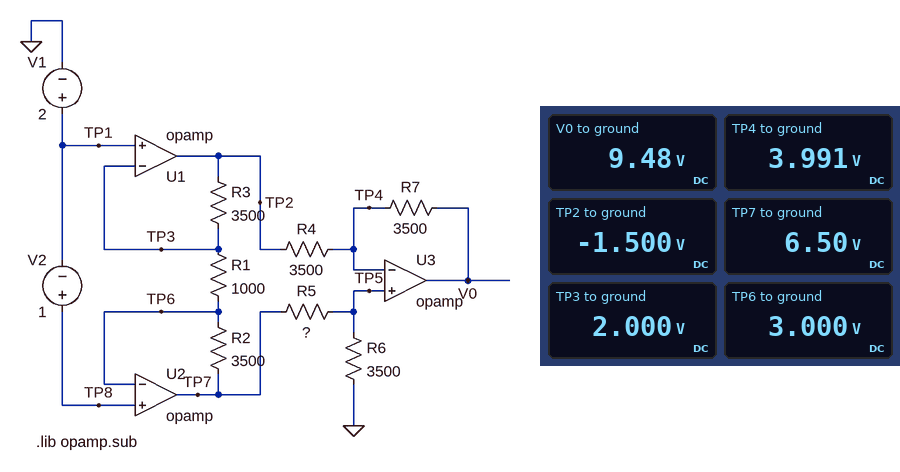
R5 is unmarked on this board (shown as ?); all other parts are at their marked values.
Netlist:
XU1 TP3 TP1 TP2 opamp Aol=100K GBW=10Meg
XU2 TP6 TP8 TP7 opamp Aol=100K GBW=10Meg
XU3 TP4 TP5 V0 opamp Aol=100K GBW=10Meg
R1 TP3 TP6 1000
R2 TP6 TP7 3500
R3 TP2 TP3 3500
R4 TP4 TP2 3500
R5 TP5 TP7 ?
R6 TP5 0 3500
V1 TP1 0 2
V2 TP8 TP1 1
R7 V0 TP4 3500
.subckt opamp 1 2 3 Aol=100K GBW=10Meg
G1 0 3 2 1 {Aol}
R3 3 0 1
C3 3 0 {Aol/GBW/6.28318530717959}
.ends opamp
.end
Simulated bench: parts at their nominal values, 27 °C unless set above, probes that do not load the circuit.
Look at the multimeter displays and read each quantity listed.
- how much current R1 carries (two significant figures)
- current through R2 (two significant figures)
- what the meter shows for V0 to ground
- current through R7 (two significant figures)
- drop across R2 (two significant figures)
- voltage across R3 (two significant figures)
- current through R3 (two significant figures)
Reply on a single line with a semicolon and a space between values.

1.0 mA; 1.0 mA; 9.48 V; 1.6 mA; 3.5 V; 3.5 V; 1.0 mA
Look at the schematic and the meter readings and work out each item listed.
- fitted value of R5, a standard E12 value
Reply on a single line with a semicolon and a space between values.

2.2 kΩ
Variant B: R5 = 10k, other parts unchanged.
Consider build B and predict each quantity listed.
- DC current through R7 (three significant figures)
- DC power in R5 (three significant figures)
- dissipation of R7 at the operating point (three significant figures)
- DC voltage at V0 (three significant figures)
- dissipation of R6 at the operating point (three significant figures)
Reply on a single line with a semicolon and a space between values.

910 µA; 2.32 mW; 2.90 mW; 4.87 V; 811 µW
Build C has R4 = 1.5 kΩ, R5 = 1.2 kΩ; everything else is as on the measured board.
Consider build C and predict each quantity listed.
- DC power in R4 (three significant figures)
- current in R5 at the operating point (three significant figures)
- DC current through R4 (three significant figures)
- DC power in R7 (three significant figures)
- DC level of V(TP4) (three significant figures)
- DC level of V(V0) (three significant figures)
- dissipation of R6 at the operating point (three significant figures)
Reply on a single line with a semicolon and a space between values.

26.8 mW; 1.38 mA; 4.23 mA; 62.5 mW; 4.84 V; 19.6 V; 6.69 mW
